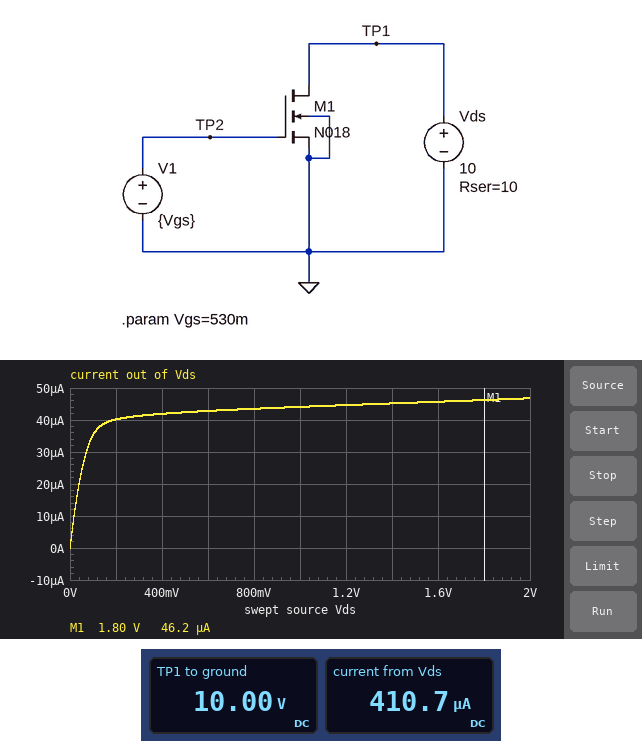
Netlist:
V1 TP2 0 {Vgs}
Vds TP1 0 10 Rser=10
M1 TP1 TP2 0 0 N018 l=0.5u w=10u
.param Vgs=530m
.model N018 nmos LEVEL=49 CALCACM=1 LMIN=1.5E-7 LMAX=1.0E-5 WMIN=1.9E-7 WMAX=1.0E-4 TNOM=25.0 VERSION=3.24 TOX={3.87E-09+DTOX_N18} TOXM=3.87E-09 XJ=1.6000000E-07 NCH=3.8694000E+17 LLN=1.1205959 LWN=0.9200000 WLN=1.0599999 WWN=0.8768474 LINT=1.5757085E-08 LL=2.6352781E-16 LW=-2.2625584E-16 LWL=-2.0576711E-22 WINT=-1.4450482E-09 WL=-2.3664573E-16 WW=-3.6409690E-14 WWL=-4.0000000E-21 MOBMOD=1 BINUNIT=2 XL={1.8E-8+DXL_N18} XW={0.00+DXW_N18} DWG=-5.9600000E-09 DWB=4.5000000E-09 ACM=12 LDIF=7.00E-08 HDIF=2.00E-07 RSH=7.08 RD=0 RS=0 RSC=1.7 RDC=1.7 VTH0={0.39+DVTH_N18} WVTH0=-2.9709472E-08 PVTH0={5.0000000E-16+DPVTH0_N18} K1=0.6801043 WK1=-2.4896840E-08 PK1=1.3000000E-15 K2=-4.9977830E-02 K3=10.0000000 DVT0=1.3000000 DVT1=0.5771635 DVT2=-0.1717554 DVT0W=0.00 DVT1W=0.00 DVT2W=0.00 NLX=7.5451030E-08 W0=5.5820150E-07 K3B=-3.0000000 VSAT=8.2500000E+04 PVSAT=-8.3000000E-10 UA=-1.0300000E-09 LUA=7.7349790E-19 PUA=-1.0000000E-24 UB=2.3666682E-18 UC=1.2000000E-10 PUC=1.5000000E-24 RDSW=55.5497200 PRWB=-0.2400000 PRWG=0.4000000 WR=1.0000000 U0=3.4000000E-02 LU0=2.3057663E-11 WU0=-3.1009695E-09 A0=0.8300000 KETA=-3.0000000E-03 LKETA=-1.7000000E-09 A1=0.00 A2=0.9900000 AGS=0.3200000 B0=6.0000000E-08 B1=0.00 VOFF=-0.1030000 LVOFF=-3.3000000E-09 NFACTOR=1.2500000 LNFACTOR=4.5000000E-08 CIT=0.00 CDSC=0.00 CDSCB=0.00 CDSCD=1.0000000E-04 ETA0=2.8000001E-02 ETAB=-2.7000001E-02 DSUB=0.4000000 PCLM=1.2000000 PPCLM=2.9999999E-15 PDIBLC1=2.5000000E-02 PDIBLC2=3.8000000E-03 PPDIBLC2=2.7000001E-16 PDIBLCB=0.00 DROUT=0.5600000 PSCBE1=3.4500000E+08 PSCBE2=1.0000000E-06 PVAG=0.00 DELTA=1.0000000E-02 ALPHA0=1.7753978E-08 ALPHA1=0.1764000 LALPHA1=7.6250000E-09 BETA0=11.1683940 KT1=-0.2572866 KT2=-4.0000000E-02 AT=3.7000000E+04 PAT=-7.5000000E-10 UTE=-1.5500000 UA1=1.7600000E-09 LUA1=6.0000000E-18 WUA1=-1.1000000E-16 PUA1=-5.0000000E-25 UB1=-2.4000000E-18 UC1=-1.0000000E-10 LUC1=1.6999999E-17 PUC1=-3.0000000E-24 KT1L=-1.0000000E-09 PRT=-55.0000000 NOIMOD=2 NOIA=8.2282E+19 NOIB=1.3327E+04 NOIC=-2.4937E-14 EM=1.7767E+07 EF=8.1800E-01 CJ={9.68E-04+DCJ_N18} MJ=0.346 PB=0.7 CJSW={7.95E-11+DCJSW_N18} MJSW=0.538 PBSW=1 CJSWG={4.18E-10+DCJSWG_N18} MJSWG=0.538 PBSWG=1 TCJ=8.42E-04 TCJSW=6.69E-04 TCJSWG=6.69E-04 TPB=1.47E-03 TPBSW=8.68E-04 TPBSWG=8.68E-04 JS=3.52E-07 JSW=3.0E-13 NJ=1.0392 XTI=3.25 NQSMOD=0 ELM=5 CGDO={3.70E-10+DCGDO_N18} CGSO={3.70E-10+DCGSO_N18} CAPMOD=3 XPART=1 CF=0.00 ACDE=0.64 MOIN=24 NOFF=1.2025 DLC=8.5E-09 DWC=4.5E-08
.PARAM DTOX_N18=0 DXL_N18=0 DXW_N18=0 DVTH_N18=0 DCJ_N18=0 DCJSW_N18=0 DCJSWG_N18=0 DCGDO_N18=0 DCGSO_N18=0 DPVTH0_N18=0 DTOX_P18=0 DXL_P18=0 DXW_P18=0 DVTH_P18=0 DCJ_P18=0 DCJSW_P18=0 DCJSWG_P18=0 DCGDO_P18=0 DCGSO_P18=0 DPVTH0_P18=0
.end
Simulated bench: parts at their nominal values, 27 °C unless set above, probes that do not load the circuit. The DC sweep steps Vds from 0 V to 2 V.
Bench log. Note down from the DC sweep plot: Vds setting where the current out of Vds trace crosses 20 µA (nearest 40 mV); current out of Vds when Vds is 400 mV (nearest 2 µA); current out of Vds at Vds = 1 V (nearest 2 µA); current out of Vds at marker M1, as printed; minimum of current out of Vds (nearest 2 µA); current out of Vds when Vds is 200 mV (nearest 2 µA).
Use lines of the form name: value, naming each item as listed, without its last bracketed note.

Vds setting where the current out of Vds trace crosses 20 µA: 40 mV
current out of Vds when Vds is 400 mV: 42 µA
current out of Vds at Vds = 1 V: 44 µA
current out of Vds at marker M1, as printed: 46.2 µA
minimum of current out of Vds: 0 A
current out of Vds when Vds is 200 mV: 40 µA
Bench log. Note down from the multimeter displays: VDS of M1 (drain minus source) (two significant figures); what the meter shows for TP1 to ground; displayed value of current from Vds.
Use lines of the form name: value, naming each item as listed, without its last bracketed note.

VDS of M1 (drain minus source): 10 V
what the meter shows for TP1 to ground: 10.00 V
displayed value of current from Vds: 410.7 µA
